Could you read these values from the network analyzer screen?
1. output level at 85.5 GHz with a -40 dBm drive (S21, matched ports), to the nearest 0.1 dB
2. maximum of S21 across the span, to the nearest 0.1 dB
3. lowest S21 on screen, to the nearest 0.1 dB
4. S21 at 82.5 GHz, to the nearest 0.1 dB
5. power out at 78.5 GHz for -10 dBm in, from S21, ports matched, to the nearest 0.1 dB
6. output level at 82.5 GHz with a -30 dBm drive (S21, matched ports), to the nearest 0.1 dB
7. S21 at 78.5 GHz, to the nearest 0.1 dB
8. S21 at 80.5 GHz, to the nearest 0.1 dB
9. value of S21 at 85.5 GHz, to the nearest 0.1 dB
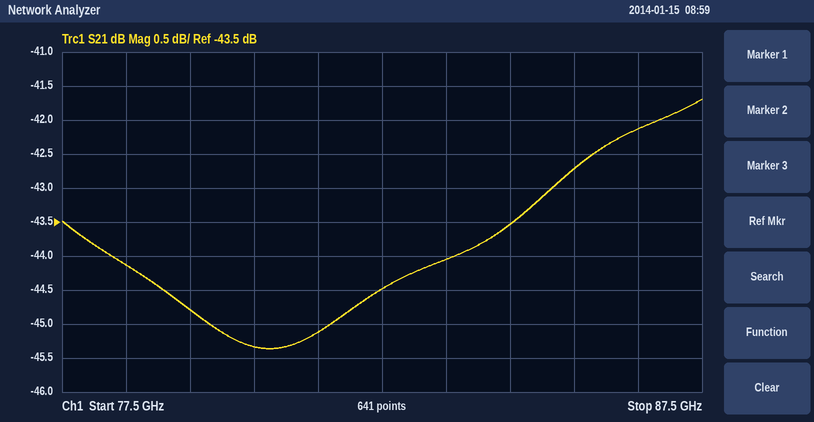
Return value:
-82.7 dBm
-41.7 dB
-45.4 dB
-44.5 dB
-54.1 dBm
-74.5 dBm
-44.1 dB
-45.3 dB
-42.7 dB
